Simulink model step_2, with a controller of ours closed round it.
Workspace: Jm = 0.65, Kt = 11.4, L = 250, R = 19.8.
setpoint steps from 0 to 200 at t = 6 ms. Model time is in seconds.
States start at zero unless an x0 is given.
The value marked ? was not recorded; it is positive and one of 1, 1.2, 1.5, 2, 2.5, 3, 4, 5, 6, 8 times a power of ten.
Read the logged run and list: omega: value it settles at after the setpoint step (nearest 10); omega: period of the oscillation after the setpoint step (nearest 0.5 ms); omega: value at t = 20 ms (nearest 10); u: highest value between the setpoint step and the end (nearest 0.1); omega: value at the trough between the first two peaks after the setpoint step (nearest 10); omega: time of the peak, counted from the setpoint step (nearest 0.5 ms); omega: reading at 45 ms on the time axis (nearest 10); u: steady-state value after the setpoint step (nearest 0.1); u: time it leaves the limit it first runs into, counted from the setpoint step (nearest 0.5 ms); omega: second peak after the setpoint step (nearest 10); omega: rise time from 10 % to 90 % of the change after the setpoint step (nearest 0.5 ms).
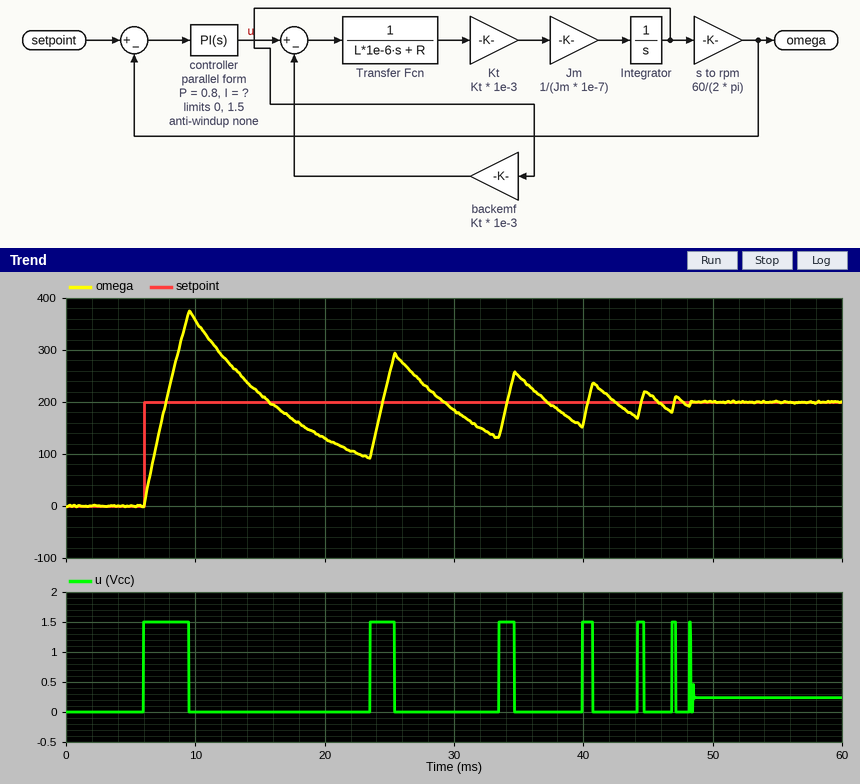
200
16.0 ms
130
1.5
90
3.5 ms
220
0.2
3.5 ms
290
1.5 ms
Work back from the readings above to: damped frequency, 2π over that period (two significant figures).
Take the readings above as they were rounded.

0.39 rad/ms
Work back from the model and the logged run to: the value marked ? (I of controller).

15000
